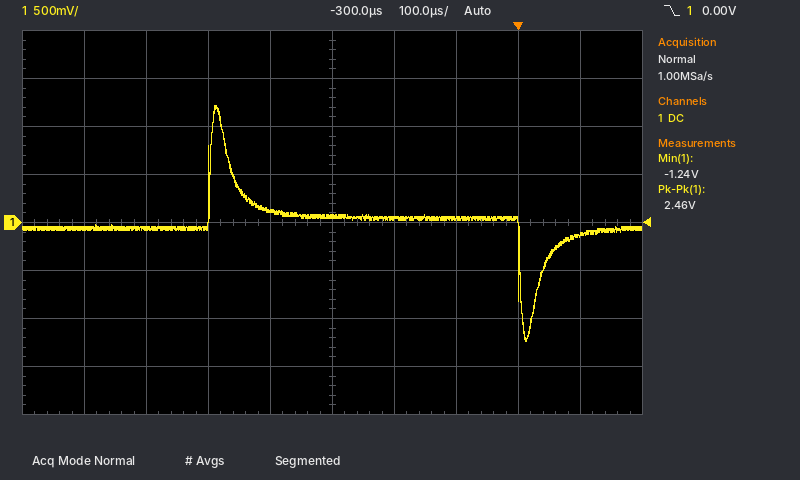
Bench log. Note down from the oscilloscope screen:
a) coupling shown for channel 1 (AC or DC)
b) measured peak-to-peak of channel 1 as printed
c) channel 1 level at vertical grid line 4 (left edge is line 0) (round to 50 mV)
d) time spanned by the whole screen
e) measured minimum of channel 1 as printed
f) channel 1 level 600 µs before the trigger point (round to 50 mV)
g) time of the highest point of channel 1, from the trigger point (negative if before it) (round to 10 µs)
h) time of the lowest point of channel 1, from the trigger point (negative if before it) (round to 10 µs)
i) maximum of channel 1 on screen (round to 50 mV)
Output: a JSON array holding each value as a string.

["DC", "2.46 V", "100 mV", "1 ms", "-1.24 V", "-50 mV", "-490 µs", "+10 µs", "1.20 V"]
